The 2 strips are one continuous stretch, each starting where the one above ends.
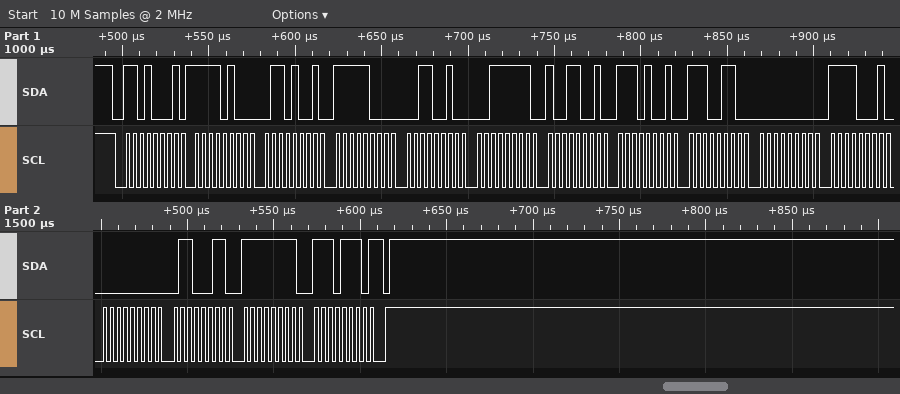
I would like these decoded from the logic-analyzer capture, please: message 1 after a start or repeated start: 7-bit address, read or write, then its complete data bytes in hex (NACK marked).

0x68 read: F4 69 F8 32 3F 99 E9 E6 00 F1 00 63 FF EE NACK
